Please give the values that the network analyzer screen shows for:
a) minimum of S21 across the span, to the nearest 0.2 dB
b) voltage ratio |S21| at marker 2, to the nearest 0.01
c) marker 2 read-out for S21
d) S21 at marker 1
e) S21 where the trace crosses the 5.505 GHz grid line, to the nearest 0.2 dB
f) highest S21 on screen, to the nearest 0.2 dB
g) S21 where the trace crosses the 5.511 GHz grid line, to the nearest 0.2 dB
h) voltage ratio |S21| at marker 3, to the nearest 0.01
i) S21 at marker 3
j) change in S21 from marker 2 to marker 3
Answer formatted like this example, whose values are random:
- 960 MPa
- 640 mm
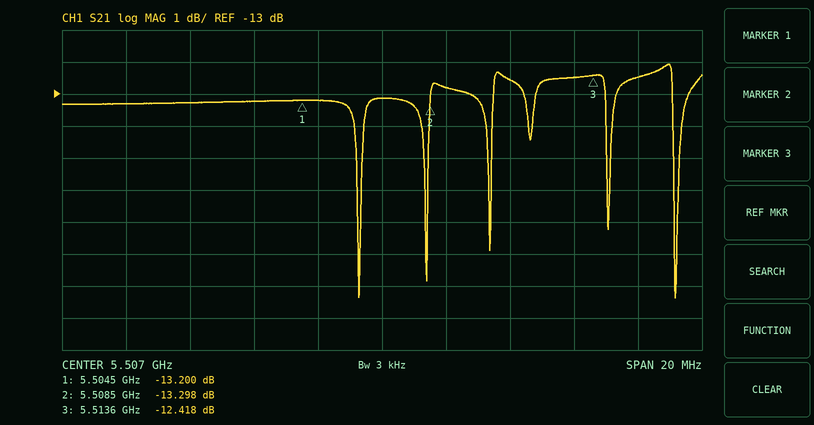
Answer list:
- -19.4 dB
- 0.22
- -13.298 dB
- -13.200 dB
- -13.2 dB
- -12.0 dB
- -12.6 dB
- 0.24
- -12.418 dB
- 0.880 dB
